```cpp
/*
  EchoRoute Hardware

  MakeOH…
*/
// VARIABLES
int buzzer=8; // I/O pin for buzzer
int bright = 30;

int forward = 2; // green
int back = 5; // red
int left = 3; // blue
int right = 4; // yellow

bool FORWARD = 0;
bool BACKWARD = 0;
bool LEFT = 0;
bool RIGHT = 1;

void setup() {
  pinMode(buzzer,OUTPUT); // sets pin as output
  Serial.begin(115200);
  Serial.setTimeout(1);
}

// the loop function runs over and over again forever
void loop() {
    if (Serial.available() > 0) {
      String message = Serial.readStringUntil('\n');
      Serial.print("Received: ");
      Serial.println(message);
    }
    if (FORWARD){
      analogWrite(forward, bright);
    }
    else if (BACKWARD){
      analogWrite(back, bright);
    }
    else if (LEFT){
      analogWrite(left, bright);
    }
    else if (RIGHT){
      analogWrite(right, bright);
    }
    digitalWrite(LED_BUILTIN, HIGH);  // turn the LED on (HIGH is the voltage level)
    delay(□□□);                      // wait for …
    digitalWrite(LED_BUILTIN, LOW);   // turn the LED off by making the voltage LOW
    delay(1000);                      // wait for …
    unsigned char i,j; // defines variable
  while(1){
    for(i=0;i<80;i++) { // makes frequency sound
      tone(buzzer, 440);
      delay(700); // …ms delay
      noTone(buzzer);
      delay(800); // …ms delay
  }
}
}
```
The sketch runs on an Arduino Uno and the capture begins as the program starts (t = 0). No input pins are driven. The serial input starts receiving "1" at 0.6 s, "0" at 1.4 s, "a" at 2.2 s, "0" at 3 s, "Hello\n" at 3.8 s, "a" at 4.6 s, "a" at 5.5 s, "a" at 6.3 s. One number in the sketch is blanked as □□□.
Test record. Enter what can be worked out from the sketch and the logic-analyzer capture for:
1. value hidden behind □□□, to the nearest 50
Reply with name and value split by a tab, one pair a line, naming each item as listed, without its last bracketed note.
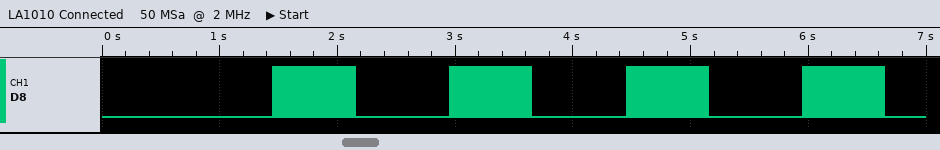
value hidden behind □□□, to the nearest 50	450
